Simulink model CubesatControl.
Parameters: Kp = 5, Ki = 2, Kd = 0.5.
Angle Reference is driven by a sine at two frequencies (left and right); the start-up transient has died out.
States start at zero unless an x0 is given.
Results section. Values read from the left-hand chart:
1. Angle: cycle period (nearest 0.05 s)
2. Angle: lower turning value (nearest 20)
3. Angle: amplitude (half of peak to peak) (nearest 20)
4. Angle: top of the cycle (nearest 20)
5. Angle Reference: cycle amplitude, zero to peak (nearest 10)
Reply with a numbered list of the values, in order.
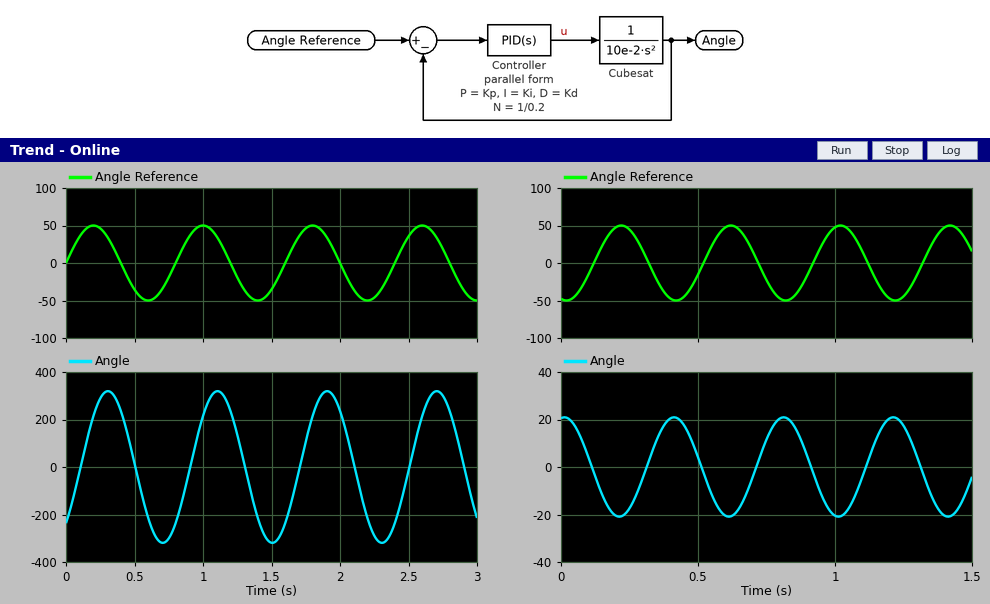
1. 0.80 s
2. -320
3. 320
4. 320
5. 50
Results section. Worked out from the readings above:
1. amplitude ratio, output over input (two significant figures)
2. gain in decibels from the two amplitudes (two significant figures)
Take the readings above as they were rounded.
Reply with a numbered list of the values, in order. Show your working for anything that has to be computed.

1. 320 / 50 = 6.4
2. 20 log10(320 / 50) = 16 dB
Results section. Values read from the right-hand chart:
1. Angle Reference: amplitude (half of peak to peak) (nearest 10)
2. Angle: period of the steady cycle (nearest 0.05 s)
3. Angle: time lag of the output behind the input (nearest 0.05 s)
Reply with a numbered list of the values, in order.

1. 50
2. 0.40 s
3. 0.20 s
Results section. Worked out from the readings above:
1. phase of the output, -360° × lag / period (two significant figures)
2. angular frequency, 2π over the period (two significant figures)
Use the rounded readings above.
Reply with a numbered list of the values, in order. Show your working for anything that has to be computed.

1. -360 × 0.2 / 0.4 = -180°
2. 2π / 0.4 = 16 rad/s
